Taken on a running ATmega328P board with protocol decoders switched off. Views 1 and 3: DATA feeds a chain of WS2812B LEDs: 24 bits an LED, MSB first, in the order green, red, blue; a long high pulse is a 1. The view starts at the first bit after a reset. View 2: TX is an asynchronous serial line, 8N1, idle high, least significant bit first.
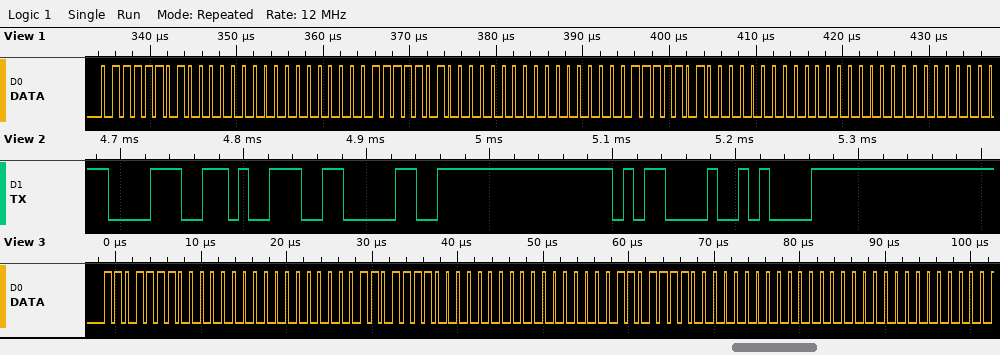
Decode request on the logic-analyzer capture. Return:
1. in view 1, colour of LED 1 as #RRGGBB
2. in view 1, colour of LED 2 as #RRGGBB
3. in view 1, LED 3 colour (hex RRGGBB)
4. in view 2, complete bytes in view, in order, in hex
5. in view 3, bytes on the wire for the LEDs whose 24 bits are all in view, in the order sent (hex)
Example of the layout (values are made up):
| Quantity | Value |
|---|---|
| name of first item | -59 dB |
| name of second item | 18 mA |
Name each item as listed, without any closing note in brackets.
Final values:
| Quantity | Value |
|---|---|
| in view 1, colour of LED 1 as #RRGGBB | #007D00 |
| in view 1, colour of LED 2 as #RRGGBB | #007D00 |
| in view 1, LED 3 colour | #007D00 |
| in view 2, complete bytes in view, in order, in hex | 38 39 30 0D 0A |
| in view 3, bytes on the wire for the LEDs whose 24 bits are all in view, in the order sent | DE 00 00 DE 00 00 DE 00 00 |
